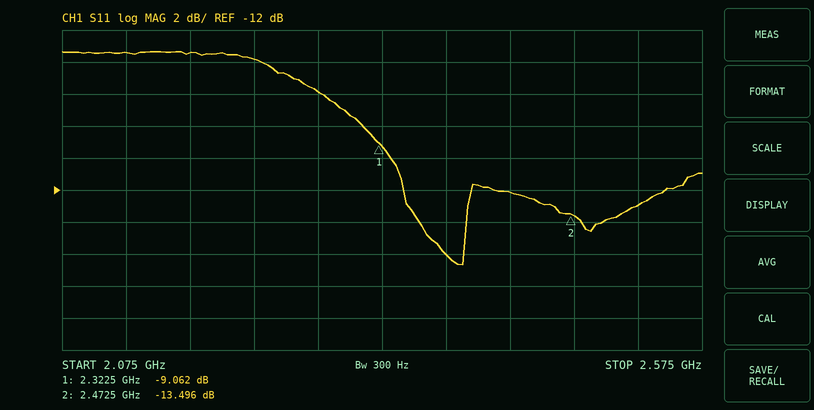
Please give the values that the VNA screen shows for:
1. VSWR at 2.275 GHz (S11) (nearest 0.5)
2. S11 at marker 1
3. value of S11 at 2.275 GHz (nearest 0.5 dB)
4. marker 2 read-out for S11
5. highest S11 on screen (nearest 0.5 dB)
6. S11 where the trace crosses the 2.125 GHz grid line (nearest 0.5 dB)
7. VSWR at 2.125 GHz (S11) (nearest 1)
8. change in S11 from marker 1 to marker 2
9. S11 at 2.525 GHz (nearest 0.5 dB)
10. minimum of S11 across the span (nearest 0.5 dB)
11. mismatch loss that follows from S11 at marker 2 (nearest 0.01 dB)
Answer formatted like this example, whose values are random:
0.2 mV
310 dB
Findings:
3.0
-9.062 dB
-6.0 dB
-13.496 dB
-3.5 dB
-3.5 dB
5
-4.434 dB
-13.0 dB
-16.5 dB
0.20 dB
